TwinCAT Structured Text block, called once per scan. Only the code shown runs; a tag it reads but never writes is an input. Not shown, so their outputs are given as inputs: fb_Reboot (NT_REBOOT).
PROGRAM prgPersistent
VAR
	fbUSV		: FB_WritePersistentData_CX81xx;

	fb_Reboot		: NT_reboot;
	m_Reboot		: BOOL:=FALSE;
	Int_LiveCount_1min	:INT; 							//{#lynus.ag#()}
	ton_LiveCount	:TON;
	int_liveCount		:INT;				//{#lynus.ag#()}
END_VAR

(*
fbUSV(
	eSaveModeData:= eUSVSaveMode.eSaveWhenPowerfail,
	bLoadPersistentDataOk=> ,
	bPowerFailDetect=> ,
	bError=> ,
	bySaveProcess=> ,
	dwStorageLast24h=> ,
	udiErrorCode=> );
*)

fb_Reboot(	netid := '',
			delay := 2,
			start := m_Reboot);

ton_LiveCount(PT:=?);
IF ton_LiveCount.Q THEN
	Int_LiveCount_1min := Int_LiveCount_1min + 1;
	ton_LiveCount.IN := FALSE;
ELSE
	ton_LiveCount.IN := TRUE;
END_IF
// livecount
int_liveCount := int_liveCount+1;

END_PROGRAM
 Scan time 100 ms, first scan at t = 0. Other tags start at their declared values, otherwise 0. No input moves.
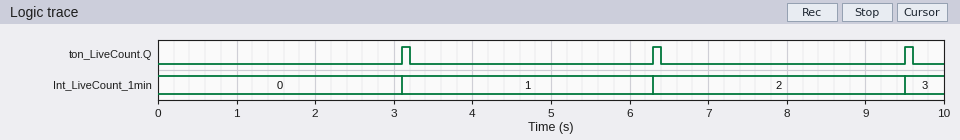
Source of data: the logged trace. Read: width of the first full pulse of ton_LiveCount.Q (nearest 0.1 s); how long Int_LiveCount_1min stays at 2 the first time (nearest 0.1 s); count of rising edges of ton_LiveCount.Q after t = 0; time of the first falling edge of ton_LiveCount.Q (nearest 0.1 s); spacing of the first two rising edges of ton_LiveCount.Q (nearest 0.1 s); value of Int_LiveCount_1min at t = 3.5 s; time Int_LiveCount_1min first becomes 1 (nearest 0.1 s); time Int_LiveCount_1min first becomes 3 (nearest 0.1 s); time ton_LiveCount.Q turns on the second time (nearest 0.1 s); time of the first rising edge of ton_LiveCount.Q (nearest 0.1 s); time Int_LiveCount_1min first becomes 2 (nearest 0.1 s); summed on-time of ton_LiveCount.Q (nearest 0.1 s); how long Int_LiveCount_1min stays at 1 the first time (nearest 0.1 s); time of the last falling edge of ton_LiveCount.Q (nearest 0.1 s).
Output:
0.1 s
3.2 s
3
3.2 s
3.2 s
1
3.1 s
9.5 s
6.3 s
3.1 s
6.3 s
0.3 s
3.2 s
9.6 s
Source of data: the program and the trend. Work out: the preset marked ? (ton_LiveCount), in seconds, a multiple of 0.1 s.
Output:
3.0 s
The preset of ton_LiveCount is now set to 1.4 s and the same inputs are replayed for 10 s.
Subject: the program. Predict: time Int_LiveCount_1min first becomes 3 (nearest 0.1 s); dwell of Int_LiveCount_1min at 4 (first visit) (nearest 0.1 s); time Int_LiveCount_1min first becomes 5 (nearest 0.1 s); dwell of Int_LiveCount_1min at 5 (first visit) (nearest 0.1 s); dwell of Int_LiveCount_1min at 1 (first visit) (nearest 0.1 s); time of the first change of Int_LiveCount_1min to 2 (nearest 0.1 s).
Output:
4.7 s
1.6 s
7.9 s
1.6 s
1.6 s
3.1 s
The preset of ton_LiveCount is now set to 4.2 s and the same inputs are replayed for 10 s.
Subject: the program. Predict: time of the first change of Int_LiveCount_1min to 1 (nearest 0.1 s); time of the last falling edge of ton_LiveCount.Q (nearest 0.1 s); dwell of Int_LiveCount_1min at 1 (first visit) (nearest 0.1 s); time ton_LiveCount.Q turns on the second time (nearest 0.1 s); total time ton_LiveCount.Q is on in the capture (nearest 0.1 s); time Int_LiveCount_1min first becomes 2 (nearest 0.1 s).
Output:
4.3 s
8.8 s
4.4 s
8.7 s
0.2 s
8.7 s
